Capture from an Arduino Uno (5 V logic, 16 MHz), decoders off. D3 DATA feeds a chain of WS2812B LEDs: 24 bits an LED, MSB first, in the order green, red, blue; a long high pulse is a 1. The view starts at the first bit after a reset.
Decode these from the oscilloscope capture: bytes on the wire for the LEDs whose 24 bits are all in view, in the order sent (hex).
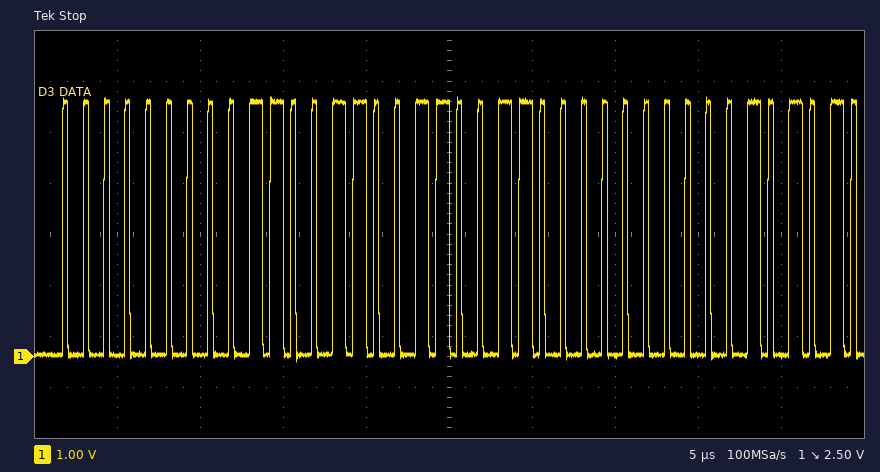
00 66 66
